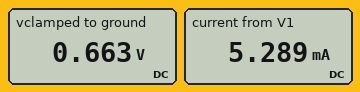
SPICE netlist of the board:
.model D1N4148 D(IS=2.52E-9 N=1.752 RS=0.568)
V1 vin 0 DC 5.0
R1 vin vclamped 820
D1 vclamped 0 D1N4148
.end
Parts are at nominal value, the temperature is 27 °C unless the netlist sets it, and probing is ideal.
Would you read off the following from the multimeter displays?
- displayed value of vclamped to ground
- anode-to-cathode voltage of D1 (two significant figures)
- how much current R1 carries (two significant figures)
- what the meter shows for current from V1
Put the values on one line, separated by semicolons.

0.663 V; 660 mV; 5.3 mA; 5.289 mA
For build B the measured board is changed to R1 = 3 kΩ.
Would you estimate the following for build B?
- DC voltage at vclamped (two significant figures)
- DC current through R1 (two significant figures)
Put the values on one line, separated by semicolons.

600 mV; 1.5 mA
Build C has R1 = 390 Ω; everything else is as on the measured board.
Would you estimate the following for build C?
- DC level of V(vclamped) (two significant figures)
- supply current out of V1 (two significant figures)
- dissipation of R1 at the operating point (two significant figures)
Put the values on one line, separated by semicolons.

700 mV; 11 mA; 47 mW
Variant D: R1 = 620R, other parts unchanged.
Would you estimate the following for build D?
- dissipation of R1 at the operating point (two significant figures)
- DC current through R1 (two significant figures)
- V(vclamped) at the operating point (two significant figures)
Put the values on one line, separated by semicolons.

30 mW; 7.0 mA; 680 mV
